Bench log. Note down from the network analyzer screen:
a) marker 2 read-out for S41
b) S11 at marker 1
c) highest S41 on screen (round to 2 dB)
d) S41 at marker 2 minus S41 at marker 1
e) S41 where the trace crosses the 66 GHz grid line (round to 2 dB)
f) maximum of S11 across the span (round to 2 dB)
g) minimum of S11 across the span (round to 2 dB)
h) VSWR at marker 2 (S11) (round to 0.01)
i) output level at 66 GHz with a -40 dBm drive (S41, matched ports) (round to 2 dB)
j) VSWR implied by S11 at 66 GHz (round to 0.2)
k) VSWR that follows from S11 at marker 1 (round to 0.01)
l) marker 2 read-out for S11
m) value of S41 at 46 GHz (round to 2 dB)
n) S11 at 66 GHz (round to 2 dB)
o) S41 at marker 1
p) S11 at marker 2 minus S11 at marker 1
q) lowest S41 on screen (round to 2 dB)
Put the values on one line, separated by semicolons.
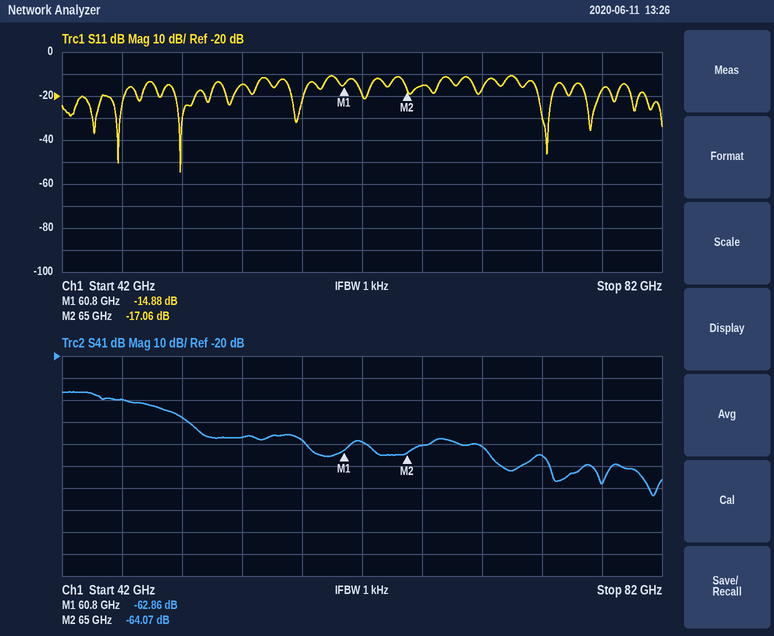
-64.07 dB; -14.88 dB; -36 dB; -1.21 dB; -60 dB; -10 dB; -54 dB; 1.33; -100 dBm; 1.4; 1.44; -17.06 dB; -40 dB; -16 dB; -62.86 dB; -2.18 dB; -84 dB
